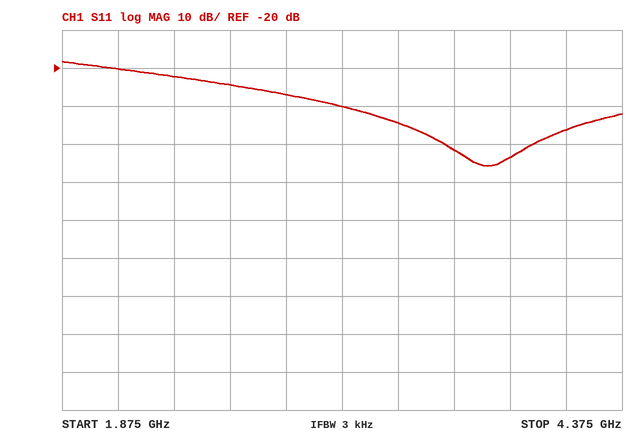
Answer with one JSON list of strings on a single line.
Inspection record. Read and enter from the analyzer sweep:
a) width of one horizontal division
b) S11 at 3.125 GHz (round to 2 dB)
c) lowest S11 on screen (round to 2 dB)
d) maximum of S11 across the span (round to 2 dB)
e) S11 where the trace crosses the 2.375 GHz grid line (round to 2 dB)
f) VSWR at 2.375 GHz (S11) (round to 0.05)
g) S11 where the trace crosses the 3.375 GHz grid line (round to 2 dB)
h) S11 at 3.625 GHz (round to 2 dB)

["250 MHz", "-30 dB", "-46 dB", "-18 dB", "-22 dB", "1.15", "-34 dB", "-42 dB"]
